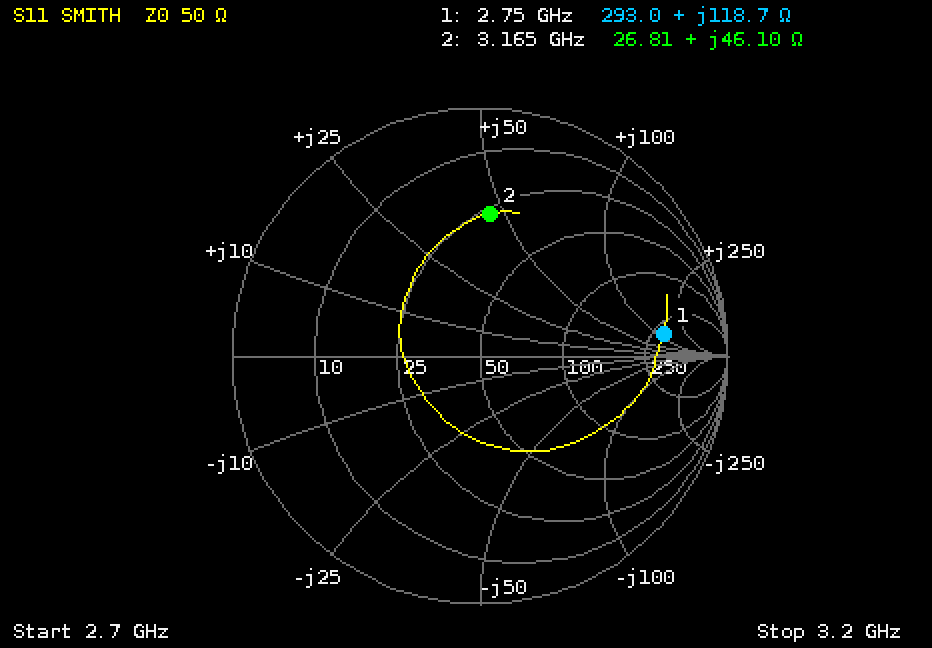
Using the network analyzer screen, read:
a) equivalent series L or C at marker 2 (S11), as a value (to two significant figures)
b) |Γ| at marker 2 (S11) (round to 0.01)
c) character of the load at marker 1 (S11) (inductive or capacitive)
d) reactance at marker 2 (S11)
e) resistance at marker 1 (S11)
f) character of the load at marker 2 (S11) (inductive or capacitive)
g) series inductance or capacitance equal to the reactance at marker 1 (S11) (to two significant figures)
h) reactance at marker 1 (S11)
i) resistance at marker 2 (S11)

2.3 nH
0.58
inductive
+46.10 Ω
293.0 Ω
inductive
6.9 nH
+118.7 Ω
26.81 Ω
